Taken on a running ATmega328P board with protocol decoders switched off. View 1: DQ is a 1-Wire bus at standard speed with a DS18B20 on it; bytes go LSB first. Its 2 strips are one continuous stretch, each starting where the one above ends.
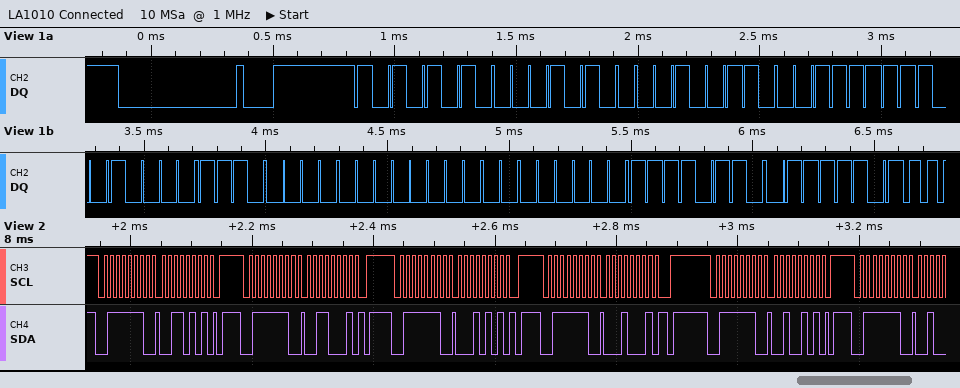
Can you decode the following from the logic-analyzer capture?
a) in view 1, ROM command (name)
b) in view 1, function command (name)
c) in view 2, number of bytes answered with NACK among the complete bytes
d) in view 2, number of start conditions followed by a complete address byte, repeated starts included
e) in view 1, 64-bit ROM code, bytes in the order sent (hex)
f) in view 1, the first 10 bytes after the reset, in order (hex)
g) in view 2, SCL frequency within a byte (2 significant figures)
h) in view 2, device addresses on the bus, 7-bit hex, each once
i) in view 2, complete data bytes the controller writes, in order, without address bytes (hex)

Match ROM
Read Scratchpad
0
6
28 64 FC 09 07 00 00 6F
55 28 64 FC 09 07 00 00 6F BE
100 kHz
0x3F
35 31 15 11 25
